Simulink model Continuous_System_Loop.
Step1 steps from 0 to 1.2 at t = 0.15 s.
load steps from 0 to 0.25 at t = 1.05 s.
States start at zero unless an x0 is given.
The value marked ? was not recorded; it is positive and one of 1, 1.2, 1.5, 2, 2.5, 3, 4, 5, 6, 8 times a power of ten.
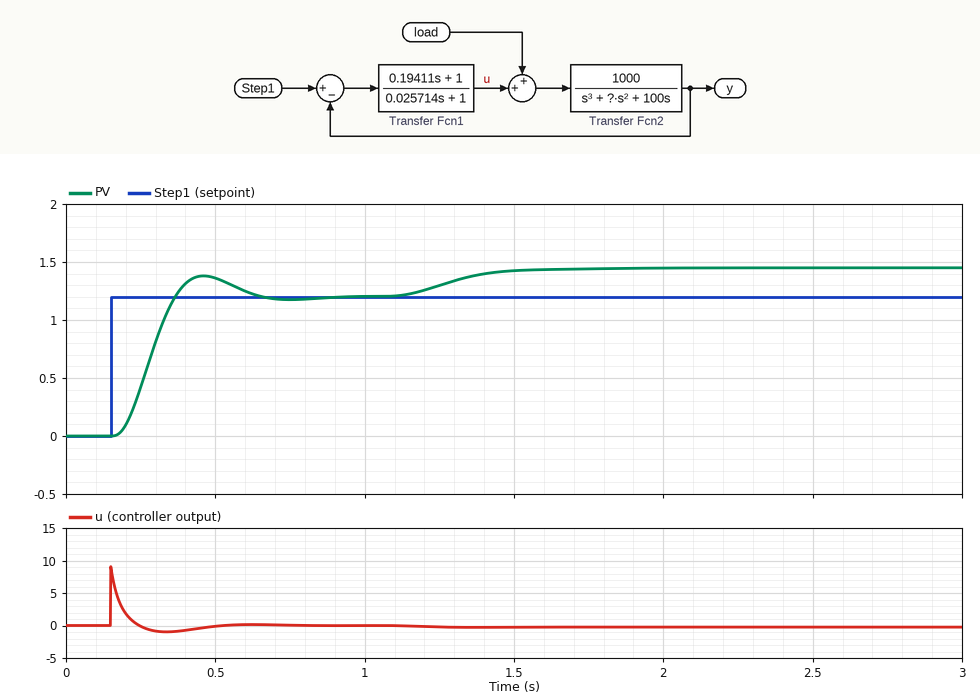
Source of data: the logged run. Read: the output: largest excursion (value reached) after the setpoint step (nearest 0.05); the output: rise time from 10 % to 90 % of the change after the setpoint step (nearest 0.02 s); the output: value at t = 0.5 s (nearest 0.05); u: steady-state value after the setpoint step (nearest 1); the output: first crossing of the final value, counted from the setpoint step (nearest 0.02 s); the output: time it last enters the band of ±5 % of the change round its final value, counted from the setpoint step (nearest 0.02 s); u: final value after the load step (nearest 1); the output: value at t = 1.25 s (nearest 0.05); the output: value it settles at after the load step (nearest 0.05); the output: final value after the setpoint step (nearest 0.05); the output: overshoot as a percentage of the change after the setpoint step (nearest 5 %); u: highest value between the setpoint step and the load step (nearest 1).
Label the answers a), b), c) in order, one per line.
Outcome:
a) 1.40
b) 0.14 s
c) 1.35
d) 0
e) 0.22 s
f) 0.44 s
g) 0
h) 1.30
i) 1.45
j) 1.20
k) 15 %
l) 9
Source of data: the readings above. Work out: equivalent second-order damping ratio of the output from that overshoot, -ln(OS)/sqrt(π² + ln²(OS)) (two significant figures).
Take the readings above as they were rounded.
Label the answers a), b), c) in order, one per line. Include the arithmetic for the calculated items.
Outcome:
a) ln(0.15) = -1.897; 1.897 / sqrt(9.870 + 3.599) = 0.52
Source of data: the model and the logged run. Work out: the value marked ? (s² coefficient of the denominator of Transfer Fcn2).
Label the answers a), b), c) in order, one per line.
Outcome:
a) 25
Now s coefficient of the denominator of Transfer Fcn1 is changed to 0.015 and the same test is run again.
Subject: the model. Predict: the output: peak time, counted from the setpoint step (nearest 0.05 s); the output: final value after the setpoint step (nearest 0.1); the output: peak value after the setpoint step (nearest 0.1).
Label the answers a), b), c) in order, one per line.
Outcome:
a) 0.30 s
b) 1.2
c) 1.3
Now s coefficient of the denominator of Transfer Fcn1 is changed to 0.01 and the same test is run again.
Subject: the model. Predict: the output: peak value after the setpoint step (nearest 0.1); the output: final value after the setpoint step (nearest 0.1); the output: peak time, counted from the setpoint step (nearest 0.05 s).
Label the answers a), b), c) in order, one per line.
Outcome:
a) 1.3
b) 1.2
c) 0.30 s
